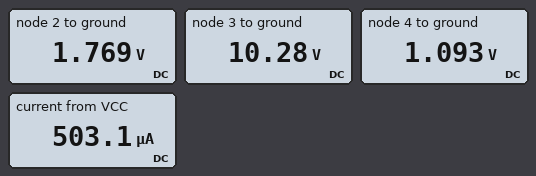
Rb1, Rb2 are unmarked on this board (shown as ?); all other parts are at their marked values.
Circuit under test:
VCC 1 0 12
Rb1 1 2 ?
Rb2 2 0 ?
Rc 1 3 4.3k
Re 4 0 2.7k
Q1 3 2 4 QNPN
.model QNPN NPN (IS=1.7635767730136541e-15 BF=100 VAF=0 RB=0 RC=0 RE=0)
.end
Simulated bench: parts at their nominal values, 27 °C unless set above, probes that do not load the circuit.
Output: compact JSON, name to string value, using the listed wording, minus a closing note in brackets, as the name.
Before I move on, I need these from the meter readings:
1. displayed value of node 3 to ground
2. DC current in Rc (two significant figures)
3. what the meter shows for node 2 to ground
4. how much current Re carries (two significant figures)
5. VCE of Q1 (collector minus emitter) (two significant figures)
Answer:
{"displayed value of node 3 to ground": "10.28 V", "DC current in Rc": "400 µA", "what the meter shows for node 2 to ground": "1.769 V", "how much current Re carries": "400 µA", "VCE of Q1 (collector minus emitter)": "9.2 V"}
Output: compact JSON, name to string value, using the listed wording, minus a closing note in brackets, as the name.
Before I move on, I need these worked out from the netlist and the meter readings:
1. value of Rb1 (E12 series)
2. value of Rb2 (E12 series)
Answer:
{"value of Rb1": "100 kΩ", "value of Rb2": "18 kΩ"}
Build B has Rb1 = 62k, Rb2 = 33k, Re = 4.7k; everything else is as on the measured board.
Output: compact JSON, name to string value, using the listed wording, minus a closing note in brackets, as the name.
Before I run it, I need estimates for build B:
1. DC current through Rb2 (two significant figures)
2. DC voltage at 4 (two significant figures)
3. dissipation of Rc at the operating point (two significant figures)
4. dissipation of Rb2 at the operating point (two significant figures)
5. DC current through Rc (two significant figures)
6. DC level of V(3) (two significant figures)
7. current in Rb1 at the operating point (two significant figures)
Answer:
{"DC current through Rb2": "120 µA", "DC voltage at 4": "3.3 V", "dissipation of Rc at the operating point": "2.1 mW", "dissipation of Rb2 at the operating point": "490 µW", "DC current through Rc": "700 µA", "DC level of V(3)": "9.0 V", "current in Rb1 at the operating point": "130 µA"}
